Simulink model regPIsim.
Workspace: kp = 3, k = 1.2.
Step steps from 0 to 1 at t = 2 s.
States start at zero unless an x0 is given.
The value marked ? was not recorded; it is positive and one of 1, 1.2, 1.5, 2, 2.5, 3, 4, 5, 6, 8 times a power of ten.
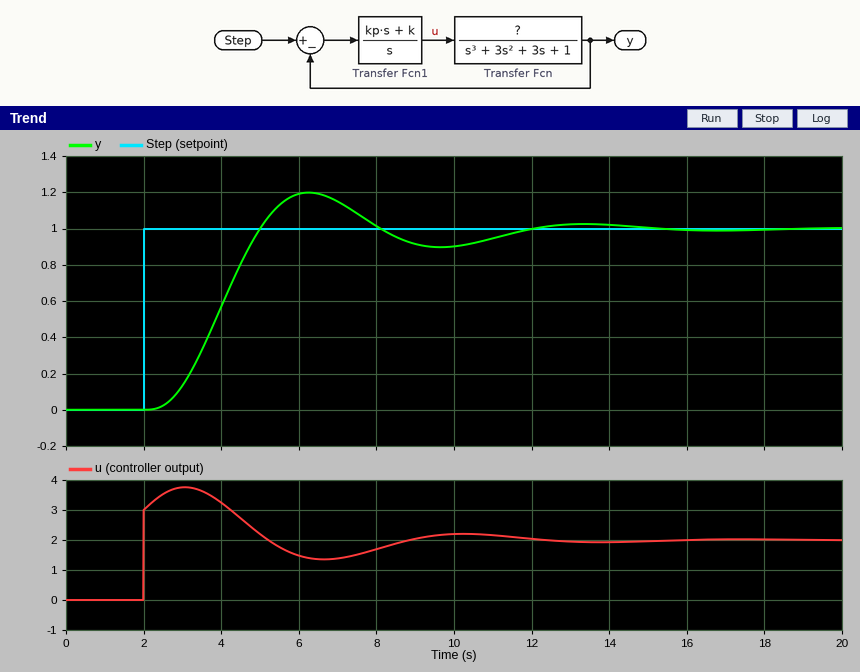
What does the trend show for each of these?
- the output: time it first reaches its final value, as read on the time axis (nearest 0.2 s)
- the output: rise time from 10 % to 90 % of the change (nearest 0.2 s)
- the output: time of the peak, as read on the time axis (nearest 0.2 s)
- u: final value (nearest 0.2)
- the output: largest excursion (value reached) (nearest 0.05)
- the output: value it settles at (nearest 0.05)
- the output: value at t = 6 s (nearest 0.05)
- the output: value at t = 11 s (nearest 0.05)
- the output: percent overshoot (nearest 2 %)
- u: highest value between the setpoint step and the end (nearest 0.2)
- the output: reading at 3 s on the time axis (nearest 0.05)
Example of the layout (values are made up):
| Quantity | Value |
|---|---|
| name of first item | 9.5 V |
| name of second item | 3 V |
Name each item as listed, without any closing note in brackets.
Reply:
| Quantity | Value |
|---|---|
| the output: time it first reaches its final value, as read on the time axis | 5.0 s |
| the output: rise time from 10 % to 90 % of the change | 1.8 s |
| the output: time of the peak, as read on the time axis | 6.2 s |
| u: final value | 2.0 |
| the output: largest excursion (value reached) | 1.20 |
| the output: value it settles at | 1.00 |
| the output: value at t = 6 s | 1.20 |
| the output: value at t = 11 s | 0.95 |
| the output: percent overshoot | 20 % |
| u: highest value between the setpoint step and the end | 3.8 |
| the output: reading at 3 s on the time axis | 0.15 |
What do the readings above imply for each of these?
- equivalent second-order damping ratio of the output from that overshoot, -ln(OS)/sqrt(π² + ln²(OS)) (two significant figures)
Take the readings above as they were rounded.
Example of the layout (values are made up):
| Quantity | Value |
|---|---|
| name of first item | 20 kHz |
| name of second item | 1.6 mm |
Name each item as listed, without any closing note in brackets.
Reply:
| Quantity | Value |
|---|---|
| equivalent second-order damping ratio of the output from that overshoot, -ln(OS)/sqrt(π² + ln²(OS)) | 0.46 |
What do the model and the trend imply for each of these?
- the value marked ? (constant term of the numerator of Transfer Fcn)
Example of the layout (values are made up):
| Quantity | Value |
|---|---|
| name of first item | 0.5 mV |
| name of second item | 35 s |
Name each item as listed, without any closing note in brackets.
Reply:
| Quantity | Value |
|---|---|
| the value marked ? | 0.5 |
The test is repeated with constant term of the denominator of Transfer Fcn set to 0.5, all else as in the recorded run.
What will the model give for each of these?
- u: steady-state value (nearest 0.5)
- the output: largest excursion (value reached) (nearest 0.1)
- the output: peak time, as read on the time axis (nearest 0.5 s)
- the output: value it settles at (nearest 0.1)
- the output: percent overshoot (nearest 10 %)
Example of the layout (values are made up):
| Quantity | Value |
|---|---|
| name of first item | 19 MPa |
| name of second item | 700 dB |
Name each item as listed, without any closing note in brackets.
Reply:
| Quantity | Value |
|---|---|
| u: steady-state value | 1.0 |
| the output: largest excursion (value reached) | 1.4 |
| the output: peak time, as read on the time axis | 6.5 s |
| the output: value it settles at | 1.0 |
| the output: percent overshoot | 40 % |
